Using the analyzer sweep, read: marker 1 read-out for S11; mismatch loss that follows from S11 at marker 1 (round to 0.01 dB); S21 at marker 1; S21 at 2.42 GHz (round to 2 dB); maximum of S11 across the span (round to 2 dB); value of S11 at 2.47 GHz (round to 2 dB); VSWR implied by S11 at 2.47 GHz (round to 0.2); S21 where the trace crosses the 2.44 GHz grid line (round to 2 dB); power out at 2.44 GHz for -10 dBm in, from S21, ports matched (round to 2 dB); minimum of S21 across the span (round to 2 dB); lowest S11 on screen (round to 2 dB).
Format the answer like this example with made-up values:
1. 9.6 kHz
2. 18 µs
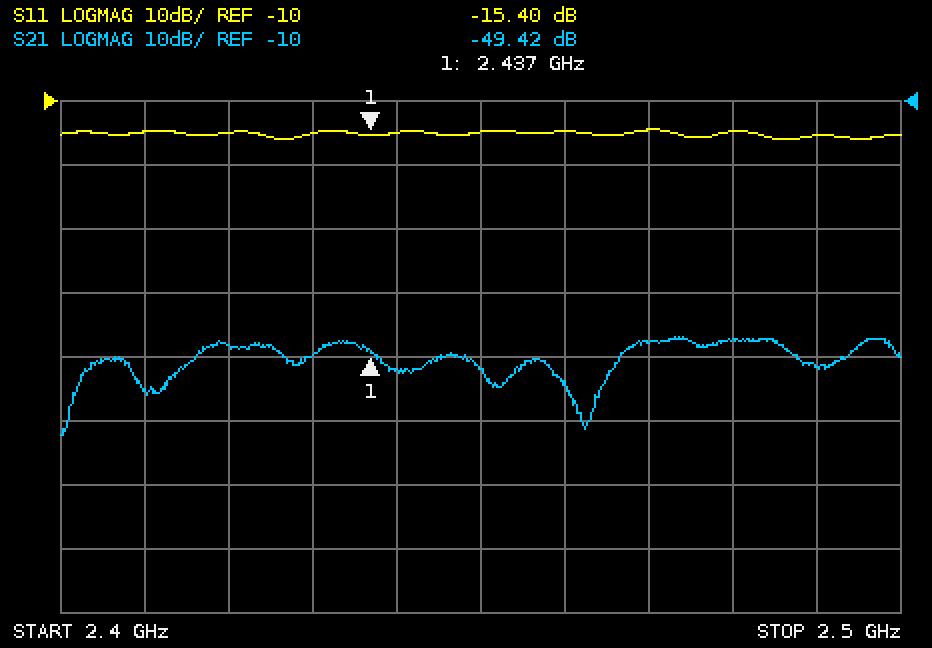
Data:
1. -15.40 dB
2. 0.13 dB
3. -49.42 dB
4. -48 dB
5. -14 dB
6. -14 dB
7. 1.4
8. -52 dB
9. -62 dBm
10. -62 dB
11. -16 dB
